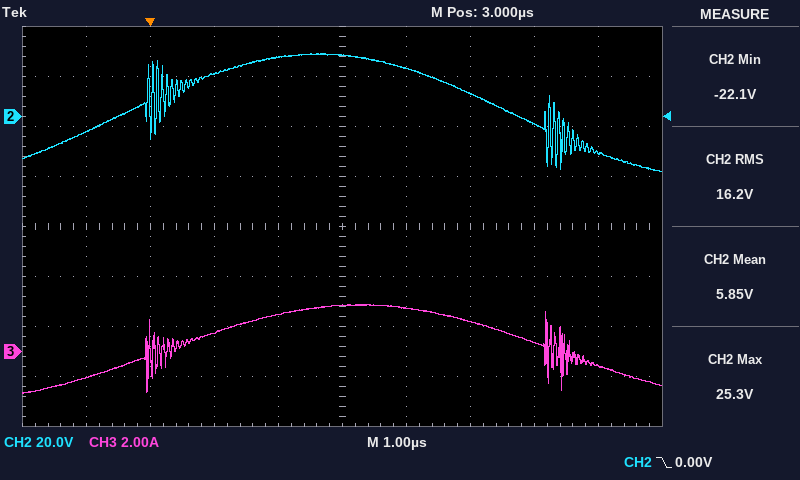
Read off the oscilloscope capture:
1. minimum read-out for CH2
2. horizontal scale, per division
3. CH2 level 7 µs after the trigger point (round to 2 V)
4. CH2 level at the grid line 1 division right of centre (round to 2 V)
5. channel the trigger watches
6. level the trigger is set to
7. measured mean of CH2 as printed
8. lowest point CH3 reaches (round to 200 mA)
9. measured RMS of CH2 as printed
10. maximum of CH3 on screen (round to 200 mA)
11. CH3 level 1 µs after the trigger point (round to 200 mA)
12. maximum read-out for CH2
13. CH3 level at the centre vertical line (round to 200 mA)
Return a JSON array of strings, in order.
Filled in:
["-22.1 V", "1 µs", "-14 V", "20 V", "CH2", "0.00 V", "5.85 V", "-1.6 A", "16.2 V", "1.8 A", "800 mA", "25.3 V", "1.8 A"]
